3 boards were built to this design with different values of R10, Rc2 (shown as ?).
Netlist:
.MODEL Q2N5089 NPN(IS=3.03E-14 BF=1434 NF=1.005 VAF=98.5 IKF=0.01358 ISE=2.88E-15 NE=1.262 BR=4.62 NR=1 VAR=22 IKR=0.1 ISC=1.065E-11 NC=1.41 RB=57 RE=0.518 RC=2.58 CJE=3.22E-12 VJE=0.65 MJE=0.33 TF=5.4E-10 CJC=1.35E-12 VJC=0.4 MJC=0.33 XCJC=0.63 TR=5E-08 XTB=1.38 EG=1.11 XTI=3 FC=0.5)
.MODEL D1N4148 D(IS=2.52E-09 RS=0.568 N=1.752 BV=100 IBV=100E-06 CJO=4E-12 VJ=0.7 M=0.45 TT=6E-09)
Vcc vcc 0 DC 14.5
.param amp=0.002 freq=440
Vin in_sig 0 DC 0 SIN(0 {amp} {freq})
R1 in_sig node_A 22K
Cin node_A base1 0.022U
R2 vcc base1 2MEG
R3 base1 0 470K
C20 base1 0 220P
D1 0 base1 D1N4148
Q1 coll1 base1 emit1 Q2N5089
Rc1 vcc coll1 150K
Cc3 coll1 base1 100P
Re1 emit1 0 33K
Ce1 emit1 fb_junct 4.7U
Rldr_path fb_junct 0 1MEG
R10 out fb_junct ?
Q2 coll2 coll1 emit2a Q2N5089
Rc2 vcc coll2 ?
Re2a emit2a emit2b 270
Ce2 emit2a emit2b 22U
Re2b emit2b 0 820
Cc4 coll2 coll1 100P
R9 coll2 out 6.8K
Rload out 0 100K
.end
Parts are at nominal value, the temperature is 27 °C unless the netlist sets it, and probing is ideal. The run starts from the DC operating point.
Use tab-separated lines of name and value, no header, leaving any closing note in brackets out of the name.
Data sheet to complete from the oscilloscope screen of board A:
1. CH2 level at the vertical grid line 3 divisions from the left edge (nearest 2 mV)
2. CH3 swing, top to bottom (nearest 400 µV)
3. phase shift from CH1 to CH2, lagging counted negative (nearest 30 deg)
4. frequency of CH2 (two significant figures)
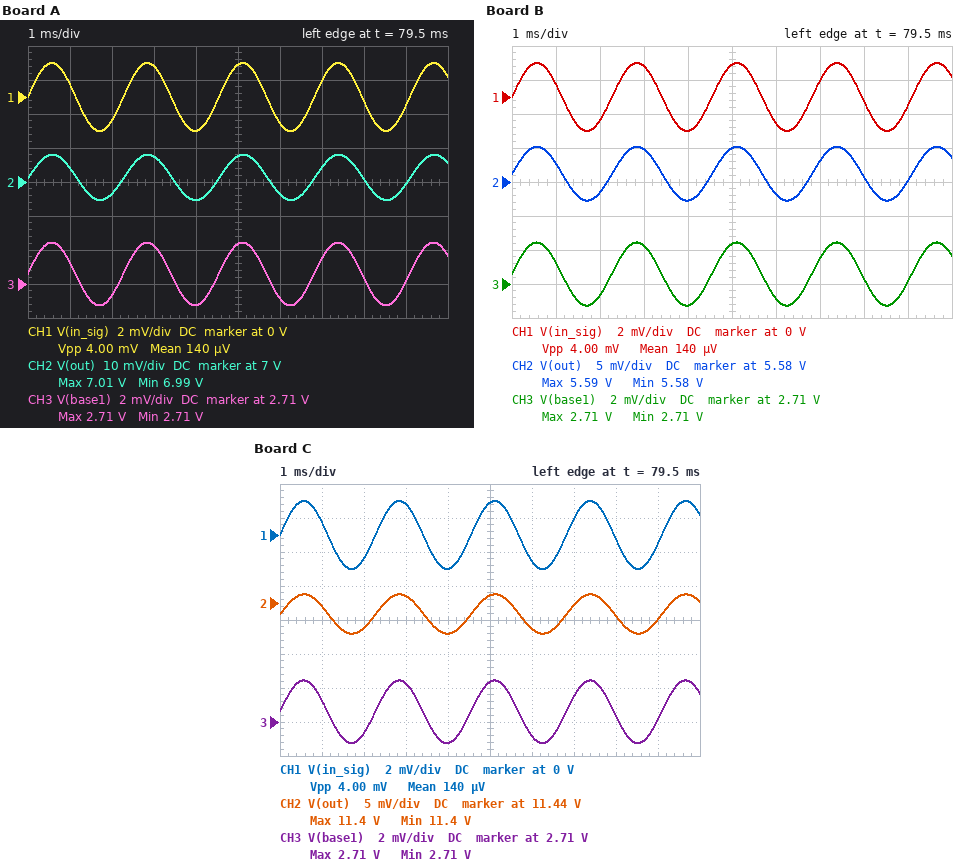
CH2 level at the vertical grid line 3 divisions from the left edge	7.008 V
CH3 swing, top to bottom	3.6 mV
phase shift from CH1 to CH2, lagging counted negative	0 deg
frequency of CH2	440 Hz
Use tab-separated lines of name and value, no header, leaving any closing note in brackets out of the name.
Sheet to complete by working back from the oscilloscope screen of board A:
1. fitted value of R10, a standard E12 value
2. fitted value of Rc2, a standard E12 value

fitted value of R10, a standard E12 value	150 kΩ
fitted value of Rc2, a standard E12 value	2.2 kΩ
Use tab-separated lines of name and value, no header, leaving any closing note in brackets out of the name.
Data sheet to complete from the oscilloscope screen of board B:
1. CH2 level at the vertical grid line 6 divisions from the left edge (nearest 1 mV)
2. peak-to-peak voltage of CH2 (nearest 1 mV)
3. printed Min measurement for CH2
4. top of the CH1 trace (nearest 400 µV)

CH2 level at the vertical grid line 6 divisions from the left edge	5.578 V
peak-to-peak voltage of CH2	8 mV
printed Min measurement for CH2	5.58 V
top of the CH1 trace	2.0 mV
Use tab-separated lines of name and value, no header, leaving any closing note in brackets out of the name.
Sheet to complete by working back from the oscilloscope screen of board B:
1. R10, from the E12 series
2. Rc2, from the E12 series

R10, from the E12 series	47 kΩ
Rc2, from the E12 series	2.7 kΩ
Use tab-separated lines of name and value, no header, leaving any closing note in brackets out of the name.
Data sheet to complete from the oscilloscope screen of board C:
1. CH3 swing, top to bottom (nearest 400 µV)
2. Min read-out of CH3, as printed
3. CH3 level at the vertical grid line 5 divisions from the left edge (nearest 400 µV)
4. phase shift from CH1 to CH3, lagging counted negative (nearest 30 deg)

CH3 swing, top to bottom	3.6 mV
Min read-out of CH3, as printed	2.71 V
CH3 level at the vertical grid line 5 divisions from the left edge	2.7124 V
phase shift from CH1 to CH3, lagging counted negative	0 deg
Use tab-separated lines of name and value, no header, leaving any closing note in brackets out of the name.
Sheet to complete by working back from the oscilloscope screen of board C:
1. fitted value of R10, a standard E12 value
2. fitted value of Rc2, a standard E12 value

fitted value of R10, a standard E12 value	47 kΩ
fitted value of Rc2, a standard E12 value	680 Ω
